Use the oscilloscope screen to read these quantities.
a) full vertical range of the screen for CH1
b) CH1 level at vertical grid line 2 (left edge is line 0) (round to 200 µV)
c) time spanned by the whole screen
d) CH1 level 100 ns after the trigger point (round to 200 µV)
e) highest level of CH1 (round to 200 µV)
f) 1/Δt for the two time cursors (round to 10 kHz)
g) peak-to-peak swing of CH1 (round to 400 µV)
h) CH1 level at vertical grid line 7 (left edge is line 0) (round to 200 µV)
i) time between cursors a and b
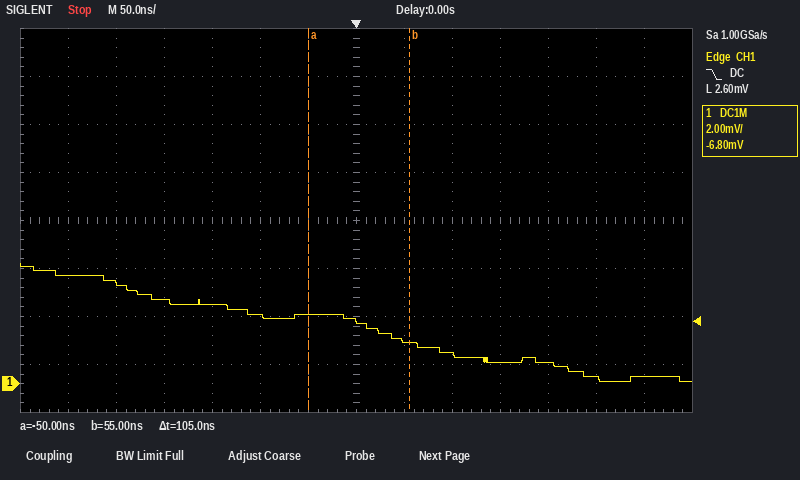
16 mV
4.2 mV
700 ns
1.2 mV
5.0 mV
9.52 MHz
4.8 mV
2.6 mV
105 ns
